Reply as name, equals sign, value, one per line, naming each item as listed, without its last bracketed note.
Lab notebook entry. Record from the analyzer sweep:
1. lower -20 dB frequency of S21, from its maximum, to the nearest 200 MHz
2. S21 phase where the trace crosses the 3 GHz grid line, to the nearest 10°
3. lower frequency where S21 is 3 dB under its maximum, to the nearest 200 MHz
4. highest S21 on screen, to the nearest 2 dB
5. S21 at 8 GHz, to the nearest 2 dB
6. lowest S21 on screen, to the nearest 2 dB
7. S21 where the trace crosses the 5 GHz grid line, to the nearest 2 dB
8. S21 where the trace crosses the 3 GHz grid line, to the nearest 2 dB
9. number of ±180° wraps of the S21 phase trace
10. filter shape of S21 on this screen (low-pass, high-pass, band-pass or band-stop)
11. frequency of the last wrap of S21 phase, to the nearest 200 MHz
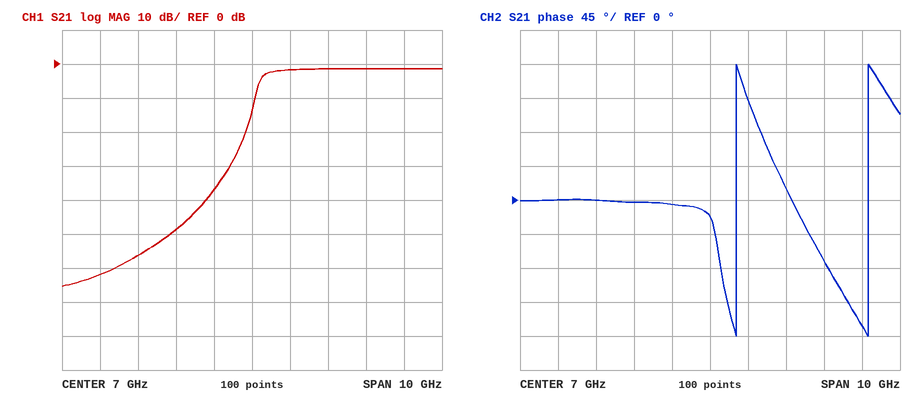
lower -20 dB frequency of S21, from its maximum, to the nearest 200 MHz = 6.8 GHz
S21 phase where the trace crosses the 3 GHz grid line, to the nearest 10° = 0°
lower frequency where S21 is 3 dB under its maximum, to the nearest 200 MHz = 7.2 GHz
highest S21 on screen, to the nearest 2 dB = -2 dB
S21 at 8 GHz, to the nearest 2 dB = -2 dB
lowest S21 on screen, to the nearest 2 dB = -66 dB
S21 where the trace crosses the 5 GHz grid line, to the nearest 2 dB = -48 dB
S21 where the trace crosses the 3 GHz grid line, to the nearest 2 dB = -62 dB
number of ±180° wraps of the S21 phase trace = 2
filter shape of S21 on this screen = high-pass
frequency of the last wrap of S21 phase, to the nearest 200 MHz = 11.2 GHz
